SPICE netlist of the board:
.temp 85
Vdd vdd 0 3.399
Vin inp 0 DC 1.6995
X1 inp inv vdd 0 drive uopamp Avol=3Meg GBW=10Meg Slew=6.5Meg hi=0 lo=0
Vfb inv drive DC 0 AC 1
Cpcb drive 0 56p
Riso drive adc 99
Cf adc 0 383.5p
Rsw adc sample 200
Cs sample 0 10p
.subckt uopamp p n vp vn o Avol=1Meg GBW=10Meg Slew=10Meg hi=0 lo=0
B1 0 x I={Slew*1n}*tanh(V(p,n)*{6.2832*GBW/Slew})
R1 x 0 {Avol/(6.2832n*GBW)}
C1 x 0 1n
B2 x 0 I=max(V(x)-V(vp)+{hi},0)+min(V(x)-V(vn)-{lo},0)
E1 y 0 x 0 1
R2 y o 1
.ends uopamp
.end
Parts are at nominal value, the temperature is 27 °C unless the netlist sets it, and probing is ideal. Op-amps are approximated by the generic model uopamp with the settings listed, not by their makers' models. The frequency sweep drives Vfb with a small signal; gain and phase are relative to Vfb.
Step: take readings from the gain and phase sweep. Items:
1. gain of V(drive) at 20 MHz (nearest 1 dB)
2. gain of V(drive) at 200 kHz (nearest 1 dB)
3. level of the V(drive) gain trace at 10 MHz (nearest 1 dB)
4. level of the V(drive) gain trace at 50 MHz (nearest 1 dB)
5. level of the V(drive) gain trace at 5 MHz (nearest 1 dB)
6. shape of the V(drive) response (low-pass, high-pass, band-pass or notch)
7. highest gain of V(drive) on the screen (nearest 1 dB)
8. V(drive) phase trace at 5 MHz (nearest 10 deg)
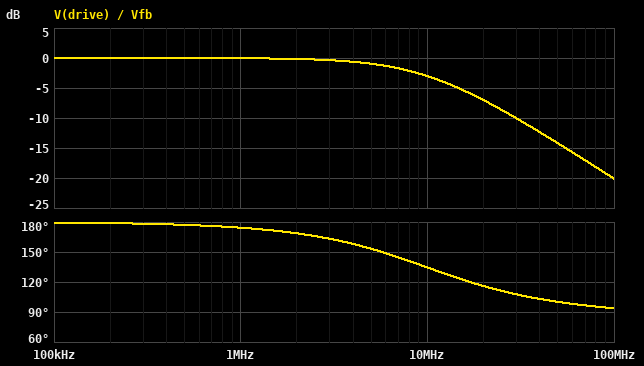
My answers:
-7 dB
0 dB
-3 dB
-14 dB
-1 dB
low-pass
0 dB
150 deg
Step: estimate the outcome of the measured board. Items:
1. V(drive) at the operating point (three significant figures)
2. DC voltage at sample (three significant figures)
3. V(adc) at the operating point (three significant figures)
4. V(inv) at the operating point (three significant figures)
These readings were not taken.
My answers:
1.70 V
1.70 V
1.70 V
1.70 V
